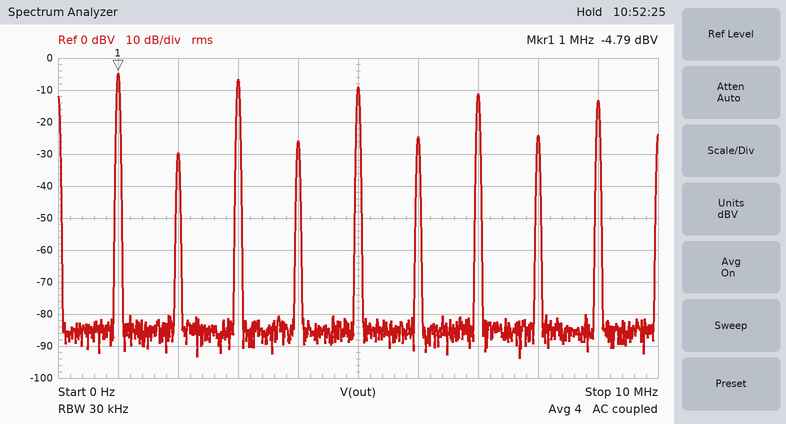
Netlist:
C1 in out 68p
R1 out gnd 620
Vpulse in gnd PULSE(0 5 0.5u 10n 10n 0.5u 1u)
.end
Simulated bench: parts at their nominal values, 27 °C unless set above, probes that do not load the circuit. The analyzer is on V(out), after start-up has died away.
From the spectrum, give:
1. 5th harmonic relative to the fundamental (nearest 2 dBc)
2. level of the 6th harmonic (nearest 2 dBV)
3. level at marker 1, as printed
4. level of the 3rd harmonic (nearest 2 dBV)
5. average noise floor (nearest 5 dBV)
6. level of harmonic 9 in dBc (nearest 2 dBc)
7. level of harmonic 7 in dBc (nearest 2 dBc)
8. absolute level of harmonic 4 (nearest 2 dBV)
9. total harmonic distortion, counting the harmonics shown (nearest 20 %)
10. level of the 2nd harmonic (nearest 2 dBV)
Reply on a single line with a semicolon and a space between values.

-4 dBc; -24 dBV; -4.79 dBV; -6 dBV; -85 dBV; -8 dBc; -6 dBc; -26 dBV; 120 %; -30 dBV
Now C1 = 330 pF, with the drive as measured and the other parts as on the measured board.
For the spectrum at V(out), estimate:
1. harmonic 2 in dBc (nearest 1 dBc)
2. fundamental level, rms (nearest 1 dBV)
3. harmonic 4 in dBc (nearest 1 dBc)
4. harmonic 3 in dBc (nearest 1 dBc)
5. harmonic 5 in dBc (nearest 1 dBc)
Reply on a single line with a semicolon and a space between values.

-29 dBc; 5 dBV; -28 dBc; -8 dBc; -12 dBc
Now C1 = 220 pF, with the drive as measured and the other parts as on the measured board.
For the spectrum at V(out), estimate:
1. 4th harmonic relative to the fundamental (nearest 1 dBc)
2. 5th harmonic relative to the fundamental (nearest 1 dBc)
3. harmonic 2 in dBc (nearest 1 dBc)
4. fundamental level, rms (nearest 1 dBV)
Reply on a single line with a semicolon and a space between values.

-27 dBc; -11 dBc; -28 dBc; 3 dBV
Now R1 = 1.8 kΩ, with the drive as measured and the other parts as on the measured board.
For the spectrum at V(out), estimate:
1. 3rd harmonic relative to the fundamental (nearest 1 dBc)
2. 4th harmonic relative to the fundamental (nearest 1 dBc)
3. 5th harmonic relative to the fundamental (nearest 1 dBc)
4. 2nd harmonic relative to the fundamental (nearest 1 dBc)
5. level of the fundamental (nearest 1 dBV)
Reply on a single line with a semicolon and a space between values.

-6 dBc; -26 dBc; -10 dBc; -27 dBc; 3 dBV
